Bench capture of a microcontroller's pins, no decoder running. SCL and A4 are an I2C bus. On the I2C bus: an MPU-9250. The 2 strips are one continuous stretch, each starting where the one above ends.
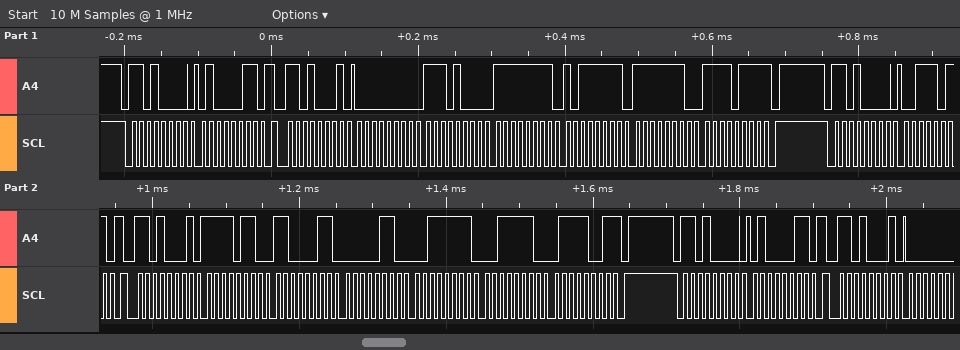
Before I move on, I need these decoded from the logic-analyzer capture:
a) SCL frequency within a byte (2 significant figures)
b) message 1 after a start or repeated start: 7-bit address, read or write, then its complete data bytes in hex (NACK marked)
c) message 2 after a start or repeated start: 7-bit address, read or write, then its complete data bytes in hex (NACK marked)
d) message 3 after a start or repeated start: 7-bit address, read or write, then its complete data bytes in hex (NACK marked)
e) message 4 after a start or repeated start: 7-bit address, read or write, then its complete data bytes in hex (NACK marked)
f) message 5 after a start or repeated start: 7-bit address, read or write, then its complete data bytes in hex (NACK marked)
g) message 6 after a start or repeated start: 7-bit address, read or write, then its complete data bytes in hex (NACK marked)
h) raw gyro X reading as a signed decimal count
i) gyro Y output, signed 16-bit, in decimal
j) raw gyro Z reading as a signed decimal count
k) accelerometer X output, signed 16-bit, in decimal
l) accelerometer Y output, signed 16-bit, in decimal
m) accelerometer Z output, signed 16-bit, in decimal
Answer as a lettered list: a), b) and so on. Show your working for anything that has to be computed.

a) 100 kHz
b) 0x68 write: 43
c) 0x68 read: 00 E8 FF BF FE F7 NACK
d) 0x68 write: 3B
e) 0x68 read: F6 C3 06 3F 3E 79 NACK
f) 0x68 write: 43
g) 0x68 read
h) 0x00E8 = 232
i) 0xFFBF = -65
j) 0xFEF7 = -265
k) 0xF6C3 = -2365
l) 0x063F = 1599
m) 0x3E79 = 15993
